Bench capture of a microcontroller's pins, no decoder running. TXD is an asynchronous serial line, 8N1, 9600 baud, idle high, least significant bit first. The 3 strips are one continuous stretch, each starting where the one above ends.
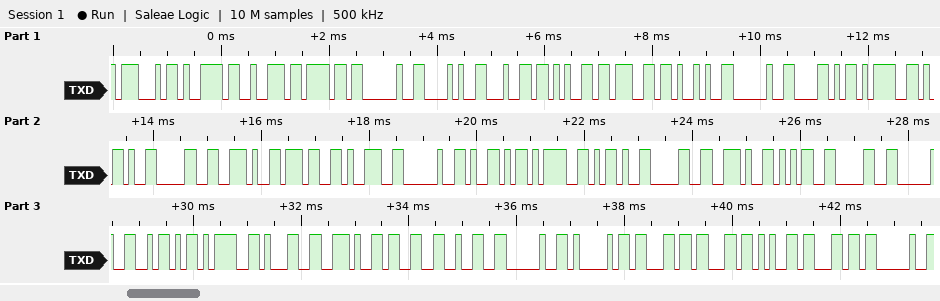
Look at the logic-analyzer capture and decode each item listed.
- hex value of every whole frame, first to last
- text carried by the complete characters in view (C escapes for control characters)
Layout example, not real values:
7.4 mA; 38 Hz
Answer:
0x47 0x79 0x72 0x6F 0x20 0x28 0x64 0x65 0x67 0x29 0x20 0x58 0x3D 0x2D 0x30 0x2E 0x37 0x39 0x20 0x59 0x3D 0x2D 0x30 0x2E 0x35 0x30 0x20 0x5A 0x3D 0x31 0x2E 0x33 0x32 0x20 0x41 0x63 0x63 0x65 0x6C 0x20; "Gyro (deg) X=-0.79 Y=-0.50 Z=1.32 Accel "
